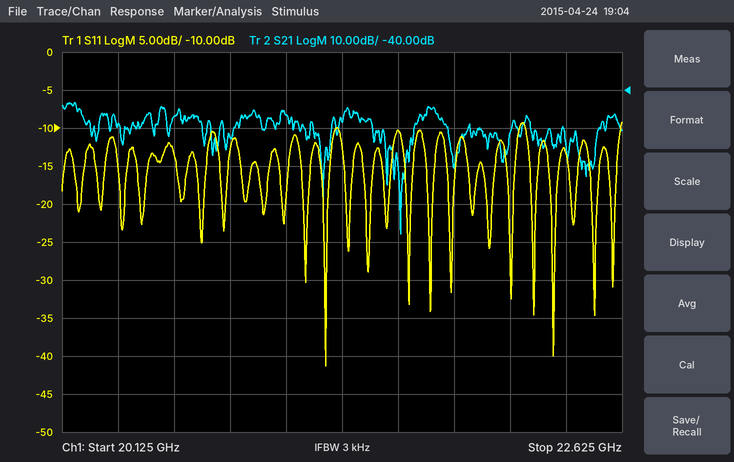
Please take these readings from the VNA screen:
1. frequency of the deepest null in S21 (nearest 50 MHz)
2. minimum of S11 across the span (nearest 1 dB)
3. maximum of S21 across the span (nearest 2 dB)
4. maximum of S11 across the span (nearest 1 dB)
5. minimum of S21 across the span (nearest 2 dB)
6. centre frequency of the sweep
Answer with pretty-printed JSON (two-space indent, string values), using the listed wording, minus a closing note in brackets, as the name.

{
  "frequency of the deepest null in S21": "21.65 GHz",
  "minimum of S11 across the span": "-41 dB",
  "maximum of S21 across the span": "-44 dB",
  "maximum of S11 across the span": "-9 dB",
  "minimum of S21 across the span": "-78 dB",
  "centre frequency of the sweep": "21.375 GHz"
}
